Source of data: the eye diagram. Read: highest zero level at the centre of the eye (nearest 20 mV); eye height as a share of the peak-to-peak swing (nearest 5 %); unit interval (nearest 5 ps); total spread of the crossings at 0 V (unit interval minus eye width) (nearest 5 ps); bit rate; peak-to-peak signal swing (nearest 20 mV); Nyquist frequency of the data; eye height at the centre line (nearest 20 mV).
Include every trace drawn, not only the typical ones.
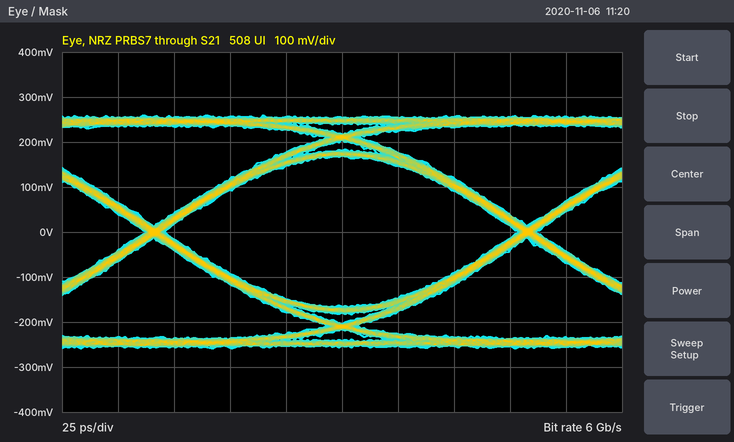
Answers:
-160 mV
65 %
165 ps
10 ps
6 Gb/s
520 mV
3 GHz
340 mV
